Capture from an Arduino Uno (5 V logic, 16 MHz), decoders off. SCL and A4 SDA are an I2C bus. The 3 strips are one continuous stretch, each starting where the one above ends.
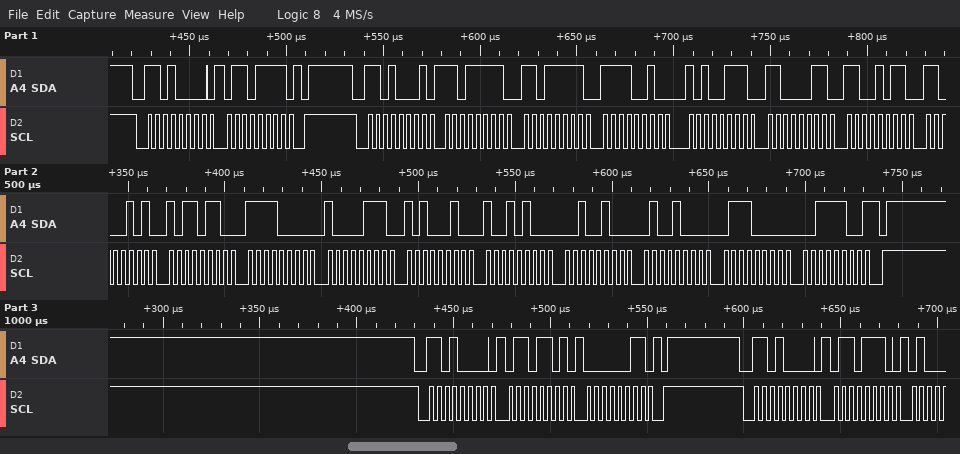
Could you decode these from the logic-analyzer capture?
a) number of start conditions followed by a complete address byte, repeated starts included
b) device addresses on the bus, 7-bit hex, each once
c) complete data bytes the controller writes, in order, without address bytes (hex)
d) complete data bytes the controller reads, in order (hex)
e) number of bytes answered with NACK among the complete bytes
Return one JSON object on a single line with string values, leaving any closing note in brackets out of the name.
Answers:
{"number of start conditions followed by a complete address byte, repeated starts included": "4", "device addresses on the bus, 7-bit hex, each once": "0x68", "complete data bytes the controller writes, in order, without address bytes": "6F 6D 03 6E", "complete data bytes the controller reads, in order": "DF DF F2 A7 C3 CB C5 B6 F0 87 A2 94 24 48 70 3C", "number of bytes answered with NACK among the complete bytes": "1"}
